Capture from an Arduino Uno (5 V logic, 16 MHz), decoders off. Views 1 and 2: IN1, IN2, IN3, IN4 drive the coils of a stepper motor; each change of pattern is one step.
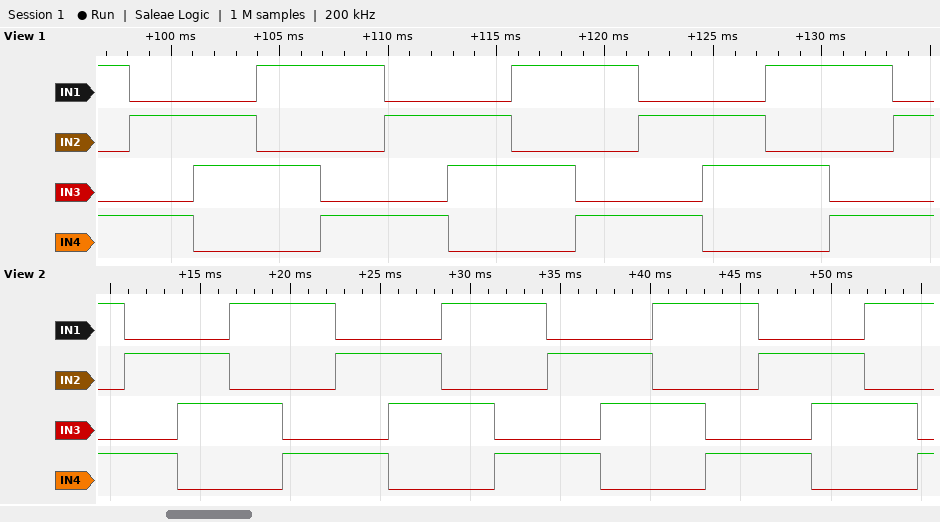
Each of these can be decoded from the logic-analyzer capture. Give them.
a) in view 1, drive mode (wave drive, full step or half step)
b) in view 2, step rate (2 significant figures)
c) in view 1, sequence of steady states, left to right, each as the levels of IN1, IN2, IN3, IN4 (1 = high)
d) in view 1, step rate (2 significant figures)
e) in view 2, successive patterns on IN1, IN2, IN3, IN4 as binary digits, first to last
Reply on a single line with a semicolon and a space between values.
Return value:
full step; 340 steps/s; 1001 0101 0110 1010 1001 0101 0110 1010 1001 0101 0110 1010 1001 0101; 340 steps/s; 1001 0101 0110 1010 1001 0101 0110 1010 1001 0101 0110 1010 1001 0101 0110 1010 1001
